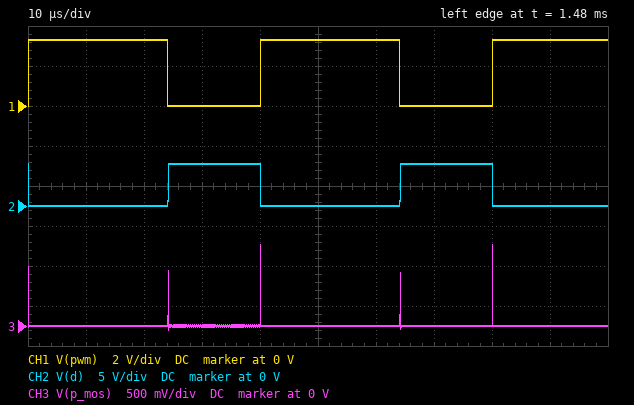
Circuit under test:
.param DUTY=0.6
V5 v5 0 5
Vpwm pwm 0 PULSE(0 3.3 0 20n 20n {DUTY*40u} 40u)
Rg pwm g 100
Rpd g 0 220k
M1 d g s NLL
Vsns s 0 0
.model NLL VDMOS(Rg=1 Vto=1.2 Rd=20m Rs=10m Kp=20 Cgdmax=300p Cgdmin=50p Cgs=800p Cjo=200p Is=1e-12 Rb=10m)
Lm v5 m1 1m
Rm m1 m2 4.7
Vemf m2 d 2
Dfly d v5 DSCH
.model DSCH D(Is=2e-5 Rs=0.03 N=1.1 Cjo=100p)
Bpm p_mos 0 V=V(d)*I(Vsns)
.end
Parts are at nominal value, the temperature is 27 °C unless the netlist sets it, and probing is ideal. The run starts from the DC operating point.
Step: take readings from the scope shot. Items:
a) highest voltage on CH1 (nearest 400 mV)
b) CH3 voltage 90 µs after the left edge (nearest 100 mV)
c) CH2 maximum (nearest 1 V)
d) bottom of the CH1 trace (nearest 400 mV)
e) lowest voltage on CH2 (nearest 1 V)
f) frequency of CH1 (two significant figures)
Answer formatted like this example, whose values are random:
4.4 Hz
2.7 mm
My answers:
3.2 V
0 V
5 V
0 V
0 V
25 kHz
